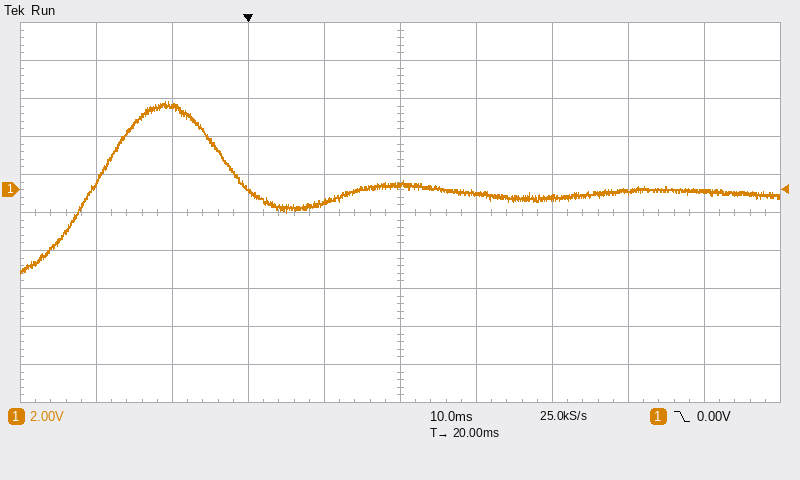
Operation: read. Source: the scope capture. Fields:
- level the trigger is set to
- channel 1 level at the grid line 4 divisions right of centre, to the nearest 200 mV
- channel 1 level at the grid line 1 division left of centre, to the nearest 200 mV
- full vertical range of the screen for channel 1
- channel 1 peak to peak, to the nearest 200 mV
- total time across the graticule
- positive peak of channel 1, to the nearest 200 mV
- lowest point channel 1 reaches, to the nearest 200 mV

0.00 V
0.0 V
-600 mV
20 V
9.0 V
100 ms
4.6 V
-4.4 V
